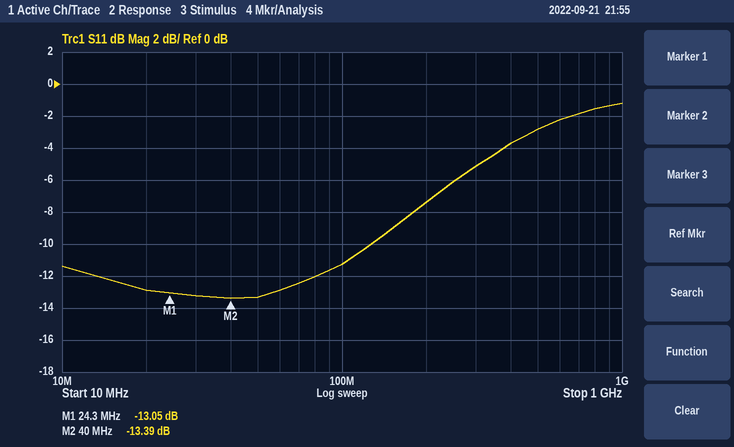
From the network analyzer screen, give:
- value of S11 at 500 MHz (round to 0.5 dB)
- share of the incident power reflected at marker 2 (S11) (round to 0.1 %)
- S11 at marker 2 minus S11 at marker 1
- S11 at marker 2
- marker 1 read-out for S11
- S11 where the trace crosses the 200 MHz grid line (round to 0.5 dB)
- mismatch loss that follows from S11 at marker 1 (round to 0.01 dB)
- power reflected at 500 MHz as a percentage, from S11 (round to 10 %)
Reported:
-3.0 dB
4.6 %
-0.34 dB
-13.39 dB
-13.05 dB
-7.5 dB
0.22 dB
50 %
